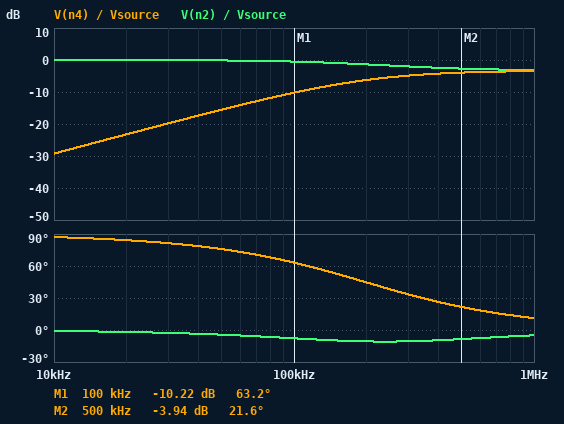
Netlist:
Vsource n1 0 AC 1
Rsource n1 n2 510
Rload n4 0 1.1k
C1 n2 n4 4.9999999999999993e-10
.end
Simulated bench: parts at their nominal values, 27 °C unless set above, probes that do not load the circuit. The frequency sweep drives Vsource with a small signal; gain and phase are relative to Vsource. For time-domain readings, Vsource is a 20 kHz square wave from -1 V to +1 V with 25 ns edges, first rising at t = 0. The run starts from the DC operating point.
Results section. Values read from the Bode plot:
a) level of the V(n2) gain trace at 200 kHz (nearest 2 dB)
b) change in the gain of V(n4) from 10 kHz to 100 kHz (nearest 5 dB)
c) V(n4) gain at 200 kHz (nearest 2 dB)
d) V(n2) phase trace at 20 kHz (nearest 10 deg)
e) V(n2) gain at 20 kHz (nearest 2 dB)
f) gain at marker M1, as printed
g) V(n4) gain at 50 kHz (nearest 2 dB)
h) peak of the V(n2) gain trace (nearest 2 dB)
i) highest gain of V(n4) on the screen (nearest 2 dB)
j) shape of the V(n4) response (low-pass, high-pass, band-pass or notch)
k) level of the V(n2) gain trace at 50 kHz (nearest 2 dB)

-2 dB
20 dB
-6 dB
0 deg
0 dB
-10.22 dB
-16 dB
0 dB
-4 dB
high-pass
0 dB
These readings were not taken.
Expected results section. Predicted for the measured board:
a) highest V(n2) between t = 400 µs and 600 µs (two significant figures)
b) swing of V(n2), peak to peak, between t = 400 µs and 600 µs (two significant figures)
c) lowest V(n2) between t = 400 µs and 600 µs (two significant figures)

1.0 V
2.0 V
-1.0 V
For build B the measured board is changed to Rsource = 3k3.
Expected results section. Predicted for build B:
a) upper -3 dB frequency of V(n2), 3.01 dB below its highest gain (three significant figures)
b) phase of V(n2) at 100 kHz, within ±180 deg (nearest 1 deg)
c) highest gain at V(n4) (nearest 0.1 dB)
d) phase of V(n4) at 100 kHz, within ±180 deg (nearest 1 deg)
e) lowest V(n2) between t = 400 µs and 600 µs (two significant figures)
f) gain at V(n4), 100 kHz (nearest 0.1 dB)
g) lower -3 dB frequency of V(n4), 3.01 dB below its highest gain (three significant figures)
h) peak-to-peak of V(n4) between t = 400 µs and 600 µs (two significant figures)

77.3 kHz
-35 deg
-12.0 dB
36 deg
-1.0 V
-13.9 dB
72.3 kHz
990 mV
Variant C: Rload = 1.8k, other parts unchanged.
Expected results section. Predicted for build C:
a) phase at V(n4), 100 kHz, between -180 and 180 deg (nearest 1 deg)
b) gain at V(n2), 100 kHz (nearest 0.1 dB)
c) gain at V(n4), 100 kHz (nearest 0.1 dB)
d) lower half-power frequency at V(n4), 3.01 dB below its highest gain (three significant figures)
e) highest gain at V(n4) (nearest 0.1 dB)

54 deg
-0.6 dB
-6.8 dB
138 kHz
-2.2 dB
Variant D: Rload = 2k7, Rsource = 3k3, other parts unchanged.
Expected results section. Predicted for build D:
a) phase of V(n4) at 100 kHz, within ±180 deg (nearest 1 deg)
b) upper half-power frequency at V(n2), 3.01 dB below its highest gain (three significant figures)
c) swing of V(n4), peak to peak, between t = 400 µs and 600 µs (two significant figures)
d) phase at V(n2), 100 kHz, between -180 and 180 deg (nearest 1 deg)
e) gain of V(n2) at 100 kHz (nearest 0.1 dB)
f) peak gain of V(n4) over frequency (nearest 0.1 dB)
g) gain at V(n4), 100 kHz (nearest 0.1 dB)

28 deg
68.8 kHz
1.8 V
-22 deg
-4.2 dB
-6.9 dB
-8.0 dB
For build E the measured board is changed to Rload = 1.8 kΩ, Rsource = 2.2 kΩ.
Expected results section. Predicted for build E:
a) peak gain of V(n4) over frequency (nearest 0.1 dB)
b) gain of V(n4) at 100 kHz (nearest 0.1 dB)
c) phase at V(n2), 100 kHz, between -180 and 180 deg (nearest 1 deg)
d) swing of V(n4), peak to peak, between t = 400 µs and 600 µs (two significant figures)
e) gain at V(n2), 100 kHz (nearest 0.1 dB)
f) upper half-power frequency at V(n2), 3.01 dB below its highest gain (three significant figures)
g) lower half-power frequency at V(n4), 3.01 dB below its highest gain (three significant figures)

-6.9 dB
-9.1 dB
-22 deg
1.8 V
-2.9 dB
103 kHz
79.6 kHz
